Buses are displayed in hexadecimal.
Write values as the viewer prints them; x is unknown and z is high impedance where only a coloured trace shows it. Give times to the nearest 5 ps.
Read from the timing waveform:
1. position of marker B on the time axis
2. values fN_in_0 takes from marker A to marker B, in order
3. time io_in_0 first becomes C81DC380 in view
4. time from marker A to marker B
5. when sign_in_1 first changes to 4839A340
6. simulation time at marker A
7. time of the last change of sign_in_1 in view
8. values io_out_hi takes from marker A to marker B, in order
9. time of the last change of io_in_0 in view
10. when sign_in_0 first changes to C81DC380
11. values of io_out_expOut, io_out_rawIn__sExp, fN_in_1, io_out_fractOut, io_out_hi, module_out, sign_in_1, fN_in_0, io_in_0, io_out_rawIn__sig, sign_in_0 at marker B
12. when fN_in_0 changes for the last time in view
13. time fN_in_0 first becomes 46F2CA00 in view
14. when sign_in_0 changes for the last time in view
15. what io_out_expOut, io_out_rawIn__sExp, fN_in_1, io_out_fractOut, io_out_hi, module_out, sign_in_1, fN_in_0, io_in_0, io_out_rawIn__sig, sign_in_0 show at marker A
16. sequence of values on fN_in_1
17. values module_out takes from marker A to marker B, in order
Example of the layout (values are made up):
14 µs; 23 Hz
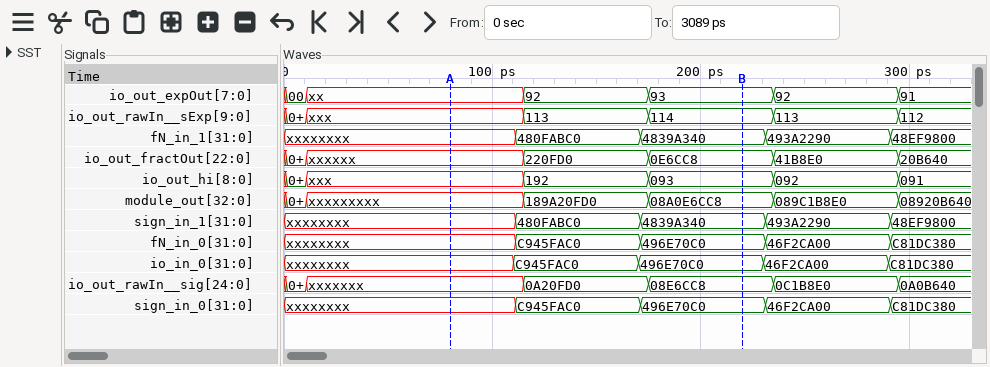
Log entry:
220 ps; xxxxxxxx, C945FAC0, 496E70C0; 290 ps; 140 ps; 170 ps; 80 ps; 290 ps; xxx, 192, 093; 290 ps; 290 ps; io_out_expOut=93, io_out_rawIn__sExp=114, fN_in_1=4839A340, io_out_fractOut=0E6CC8, io_out_hi=093, module_out=08A0E6CC8, sign_in_1=4839A340, fN_in_0=496E70C0, io_in_0=496E70C0, io_out_rawIn__sig=08E6CC8, sign_in_0=496E70C0; 290 ps; 230 ps; 290 ps; io_out_expOut=xx, io_out_rawIn__sExp=xxx, fN_in_1=xxxxxxxx, io_out_fractOut=xxxxxx, io_out_hi=xxx, module_out=xxxxxxxxx, sign_in_1=xxxxxxxx, fN_in_0=xxxxxxxx, io_in_0=xxxxxxxx, io_out_rawIn__sig=xxxxxxx, sign_in_0=xxxxxxxx; xxxxxxxx, 480FABC0, 4839A340, 493A2290, 48EF9800; xxxxxxxxx, 189A20FD0, 08A0E6CC8
